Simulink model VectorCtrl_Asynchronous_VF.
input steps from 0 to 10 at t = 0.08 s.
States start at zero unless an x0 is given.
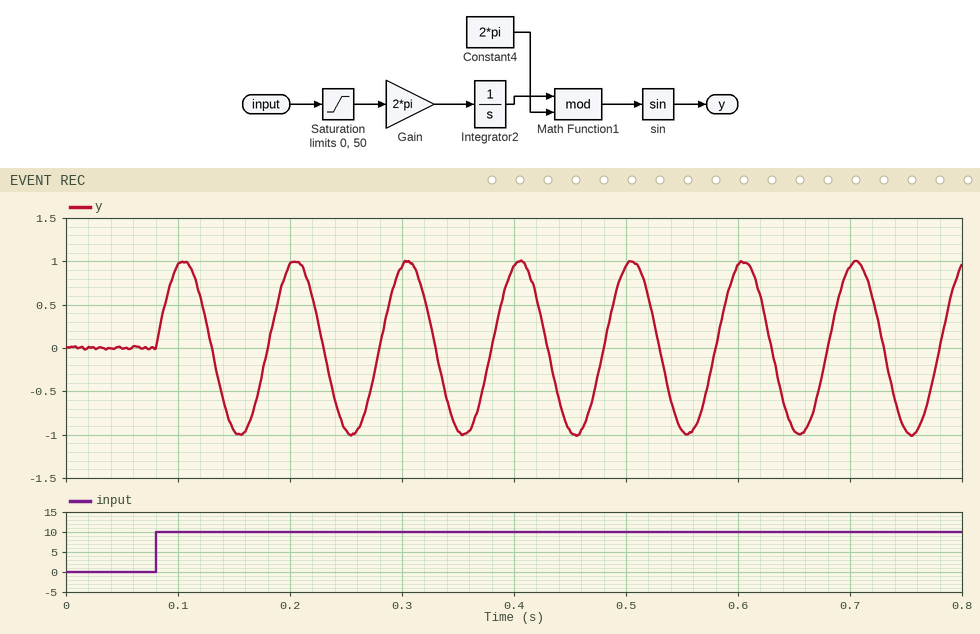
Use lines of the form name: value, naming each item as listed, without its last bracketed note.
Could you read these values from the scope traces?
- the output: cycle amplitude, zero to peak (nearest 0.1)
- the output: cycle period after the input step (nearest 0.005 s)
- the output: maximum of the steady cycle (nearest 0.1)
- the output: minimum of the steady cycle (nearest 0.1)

the output: cycle amplitude, zero to peak: 1.0
the output: cycle period after the input step: 0.100 s
the output: maximum of the steady cycle: 1.0
the output: minimum of the steady cycle: -1.0
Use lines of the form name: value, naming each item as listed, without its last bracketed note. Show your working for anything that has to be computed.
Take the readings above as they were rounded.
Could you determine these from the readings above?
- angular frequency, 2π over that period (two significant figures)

angular frequency, 2π over that period: 2π / 0.1 = 63 rad/s
